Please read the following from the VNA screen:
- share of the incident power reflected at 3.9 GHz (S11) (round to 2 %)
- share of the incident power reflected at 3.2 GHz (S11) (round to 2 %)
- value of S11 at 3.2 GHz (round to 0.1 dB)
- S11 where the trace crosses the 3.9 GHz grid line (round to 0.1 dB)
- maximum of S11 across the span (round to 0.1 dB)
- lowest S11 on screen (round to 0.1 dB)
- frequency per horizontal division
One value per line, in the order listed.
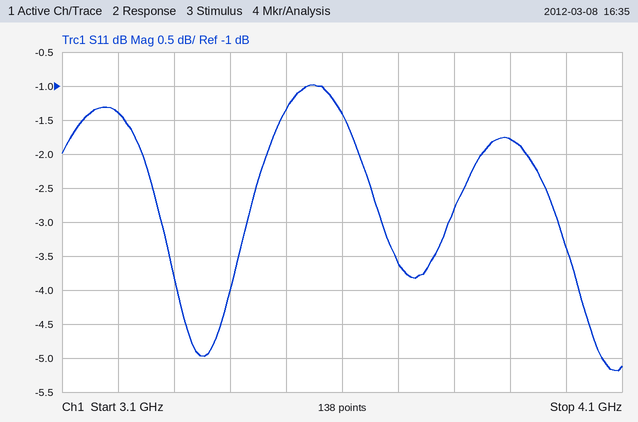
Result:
66 %
72 %
-1.4 dB
-1.8 dB
-1.0 dB
-5.2 dB
100 MHz
